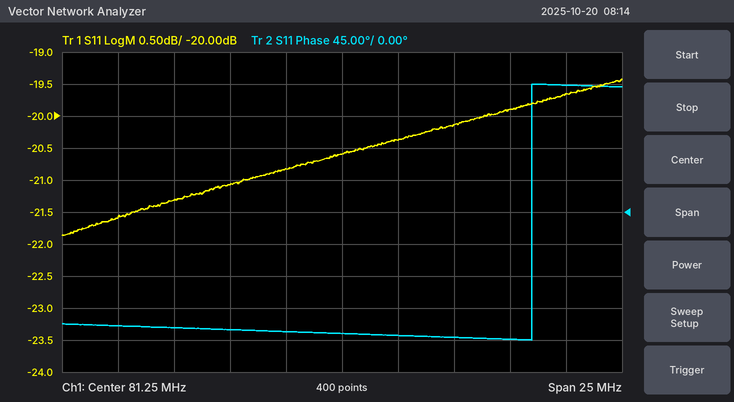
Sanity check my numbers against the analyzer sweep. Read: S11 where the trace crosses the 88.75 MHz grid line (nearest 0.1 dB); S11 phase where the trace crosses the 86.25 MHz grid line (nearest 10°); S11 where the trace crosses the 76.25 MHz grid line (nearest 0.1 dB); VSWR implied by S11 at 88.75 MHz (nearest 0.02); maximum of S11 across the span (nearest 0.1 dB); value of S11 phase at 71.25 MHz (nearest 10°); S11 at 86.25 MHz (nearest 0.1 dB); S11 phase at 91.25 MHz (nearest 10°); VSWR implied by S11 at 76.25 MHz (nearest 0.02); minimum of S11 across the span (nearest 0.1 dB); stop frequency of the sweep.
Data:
-19.9 dB
-180°
-21.1 dB
1.22
-19.4 dB
-160°
-20.1 dB
180°
1.20
-21.9 dB
93.75 MHz
